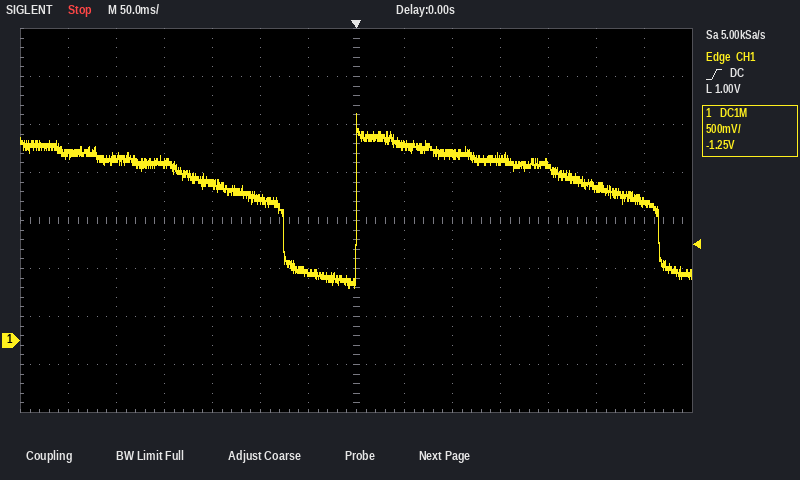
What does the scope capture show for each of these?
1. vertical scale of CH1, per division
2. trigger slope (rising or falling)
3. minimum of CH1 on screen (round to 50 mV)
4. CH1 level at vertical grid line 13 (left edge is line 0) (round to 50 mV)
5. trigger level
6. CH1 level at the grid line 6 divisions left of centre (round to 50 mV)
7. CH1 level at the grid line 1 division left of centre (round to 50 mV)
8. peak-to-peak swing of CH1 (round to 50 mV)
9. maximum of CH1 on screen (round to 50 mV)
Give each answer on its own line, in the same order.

500 mV
rising
550 mV
1.45 V
1.00 V
1.95 V
700 mV
1.80 V
2.35 V
